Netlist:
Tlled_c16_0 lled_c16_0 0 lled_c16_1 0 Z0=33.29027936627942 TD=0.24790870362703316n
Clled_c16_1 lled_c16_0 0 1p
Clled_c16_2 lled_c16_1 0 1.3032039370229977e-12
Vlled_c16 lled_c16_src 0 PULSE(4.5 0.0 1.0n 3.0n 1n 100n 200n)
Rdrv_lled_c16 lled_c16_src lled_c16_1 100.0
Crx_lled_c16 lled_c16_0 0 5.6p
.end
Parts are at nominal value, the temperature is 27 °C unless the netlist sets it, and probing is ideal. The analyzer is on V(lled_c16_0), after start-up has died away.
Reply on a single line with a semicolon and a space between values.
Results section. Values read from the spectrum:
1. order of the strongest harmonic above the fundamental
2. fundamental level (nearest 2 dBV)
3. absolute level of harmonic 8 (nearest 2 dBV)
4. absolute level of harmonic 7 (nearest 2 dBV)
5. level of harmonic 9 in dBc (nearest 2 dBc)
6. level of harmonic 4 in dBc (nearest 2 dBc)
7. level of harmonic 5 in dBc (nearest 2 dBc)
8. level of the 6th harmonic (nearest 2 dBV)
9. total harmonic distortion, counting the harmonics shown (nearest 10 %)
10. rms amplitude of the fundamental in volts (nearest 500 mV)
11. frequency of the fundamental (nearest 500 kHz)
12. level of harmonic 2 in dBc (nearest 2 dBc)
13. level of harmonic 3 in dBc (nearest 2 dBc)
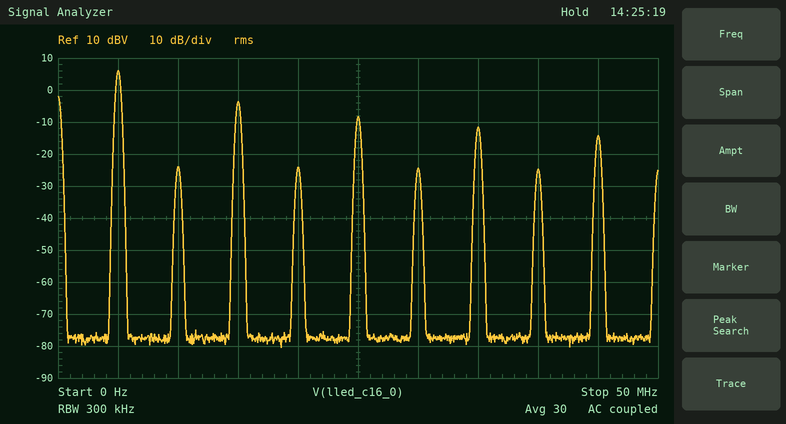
3; 6 dBV; -24 dBV; -12 dBV; -20 dBc; -30 dBc; -14 dBc; -24 dBV; 40 %; 2.0 V; 5.0 MHz; -30 dBc; -10 dBc
